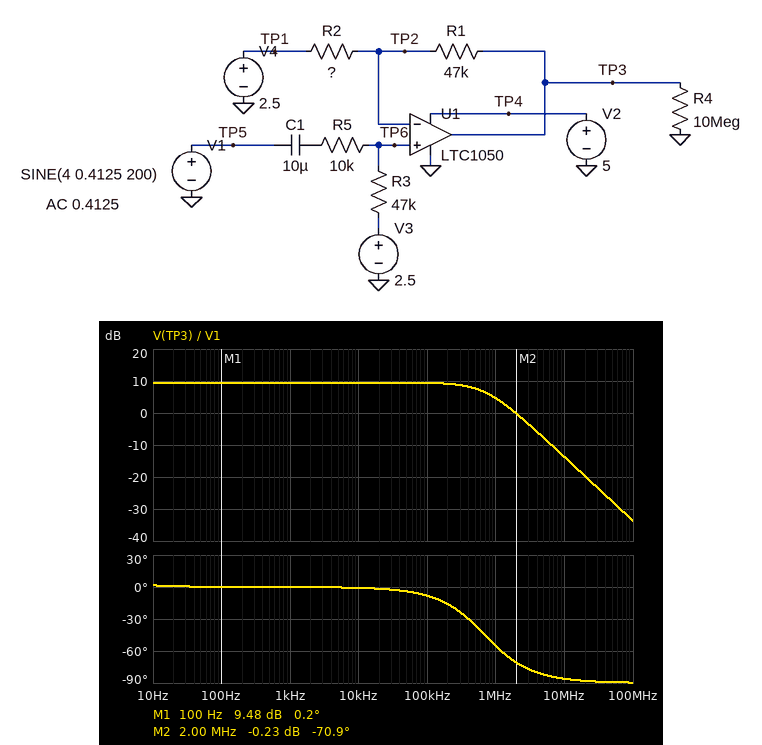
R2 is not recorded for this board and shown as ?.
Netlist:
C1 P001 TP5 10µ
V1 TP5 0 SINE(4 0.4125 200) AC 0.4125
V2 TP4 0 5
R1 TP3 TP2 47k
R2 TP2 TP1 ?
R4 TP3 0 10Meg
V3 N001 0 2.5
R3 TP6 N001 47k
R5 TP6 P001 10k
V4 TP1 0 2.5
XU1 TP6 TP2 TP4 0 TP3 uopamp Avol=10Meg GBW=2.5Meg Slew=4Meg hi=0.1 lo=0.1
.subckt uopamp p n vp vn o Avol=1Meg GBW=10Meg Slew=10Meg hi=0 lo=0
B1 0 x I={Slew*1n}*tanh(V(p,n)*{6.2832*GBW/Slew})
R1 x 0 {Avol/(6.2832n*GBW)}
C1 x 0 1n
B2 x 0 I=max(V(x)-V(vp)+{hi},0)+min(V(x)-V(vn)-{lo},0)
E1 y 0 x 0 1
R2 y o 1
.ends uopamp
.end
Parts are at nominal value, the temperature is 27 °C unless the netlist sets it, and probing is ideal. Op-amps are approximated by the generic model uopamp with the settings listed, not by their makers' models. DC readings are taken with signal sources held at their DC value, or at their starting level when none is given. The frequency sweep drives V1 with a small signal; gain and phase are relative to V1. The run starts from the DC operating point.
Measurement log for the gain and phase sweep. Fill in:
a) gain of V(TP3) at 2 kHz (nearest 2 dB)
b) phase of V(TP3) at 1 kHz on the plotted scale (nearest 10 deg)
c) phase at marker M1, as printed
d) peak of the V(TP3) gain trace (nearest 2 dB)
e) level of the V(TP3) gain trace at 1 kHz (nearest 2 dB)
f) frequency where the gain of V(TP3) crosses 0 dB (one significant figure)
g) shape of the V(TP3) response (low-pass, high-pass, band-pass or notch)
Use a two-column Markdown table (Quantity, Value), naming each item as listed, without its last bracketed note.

| Quantity | Value |
|---|---|
| gain of V(TP3) at 2 kHz | 10 dB |
| phase of V(TP3) at 1 kHz on the plotted scale | 0 deg |
| phase at marker M1, as printed | 0.2 deg |
| peak of the V(TP3) gain trace | 10 dB |
| level of the V(TP3) gain trace at 1 kHz | 10 dB |
| frequency where the gain of V(TP3) crosses 0 dB | 2 MHz |
| shape of the V(TP3) response | low-pass |
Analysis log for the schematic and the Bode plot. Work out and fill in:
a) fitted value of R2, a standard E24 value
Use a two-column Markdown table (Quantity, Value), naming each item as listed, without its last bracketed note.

| Quantity | Value |
|---|---|
| fitted value of R2, a standard E24 value | 18 kΩ |
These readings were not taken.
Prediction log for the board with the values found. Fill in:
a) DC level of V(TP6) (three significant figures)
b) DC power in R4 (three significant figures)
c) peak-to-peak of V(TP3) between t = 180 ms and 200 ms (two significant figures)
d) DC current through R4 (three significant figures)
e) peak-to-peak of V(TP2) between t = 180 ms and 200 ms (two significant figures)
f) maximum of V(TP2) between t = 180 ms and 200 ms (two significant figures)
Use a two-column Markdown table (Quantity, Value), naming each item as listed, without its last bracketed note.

| Quantity | Value |
|---|---|
| DC level of V(TP6) | 2.50 V |
| DC power in R4 | 625 nW |
| peak-to-peak of V(TP3) between t = 180 ms and 200 ms | 2.5 V |
| DC current through R4 | 250 nA |
| peak-to-peak of V(TP2) between t = 180 ms and 200 ms | 680 mV |
| maximum of V(TP2) between t = 180 ms and 200 ms | 2.8 V |
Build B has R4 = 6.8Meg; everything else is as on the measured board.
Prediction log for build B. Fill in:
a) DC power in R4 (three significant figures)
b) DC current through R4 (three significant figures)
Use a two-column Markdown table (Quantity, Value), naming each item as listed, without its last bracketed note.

| Quantity | Value |
|---|---|
| DC power in R4 | 919 nW |
| DC current through R4 | 368 nA |
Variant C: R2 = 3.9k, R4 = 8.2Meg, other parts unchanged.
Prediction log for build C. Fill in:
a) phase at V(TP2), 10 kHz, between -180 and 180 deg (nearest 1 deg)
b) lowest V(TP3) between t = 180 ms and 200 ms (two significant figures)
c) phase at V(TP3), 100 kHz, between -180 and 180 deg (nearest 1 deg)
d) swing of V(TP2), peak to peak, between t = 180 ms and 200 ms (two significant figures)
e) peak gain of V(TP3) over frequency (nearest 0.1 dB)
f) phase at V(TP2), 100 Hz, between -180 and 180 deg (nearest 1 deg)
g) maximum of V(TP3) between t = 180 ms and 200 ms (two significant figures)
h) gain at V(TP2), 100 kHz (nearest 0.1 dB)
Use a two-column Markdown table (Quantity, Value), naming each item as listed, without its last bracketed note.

| Quantity | Value |
|---|---|
| phase at V(TP2), 10 kHz, between -180 and 180 deg | -3 deg |
| lowest V(TP3) between t = 180 ms and 200 ms | 98 mV |
| phase at V(TP3), 100 kHz, between -180 and 180 deg | -28 deg |
| swing of V(TP2), peak to peak, between t = 180 ms and 200 ms | 370 mV |
| peak gain of V(TP3) over frequency | 20.6 dB |
| phase at V(TP2), 100 Hz, between -180 and 180 deg | 0 deg |
| maximum of V(TP3) between t = 180 ms and 200 ms | 4.9 V |
| gain at V(TP2), 100 kHz | -2.7 dB |
